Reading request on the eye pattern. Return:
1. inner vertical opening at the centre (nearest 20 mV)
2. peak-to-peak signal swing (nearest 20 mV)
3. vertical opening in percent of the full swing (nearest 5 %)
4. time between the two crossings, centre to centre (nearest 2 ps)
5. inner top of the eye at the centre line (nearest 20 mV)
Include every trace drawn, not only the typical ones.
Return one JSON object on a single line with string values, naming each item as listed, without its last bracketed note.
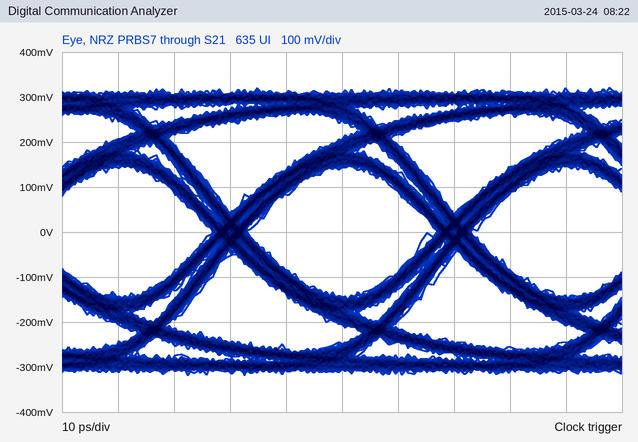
{"inner vertical opening at the centre": "280 mV", "peak-to-peak signal swing": "640 mV", "vertical opening in percent of the full swing": "45 %", "time between the two crossings, centre to centre": "40 ps", "inner top of the eye at the centre line": "140 mV"}
